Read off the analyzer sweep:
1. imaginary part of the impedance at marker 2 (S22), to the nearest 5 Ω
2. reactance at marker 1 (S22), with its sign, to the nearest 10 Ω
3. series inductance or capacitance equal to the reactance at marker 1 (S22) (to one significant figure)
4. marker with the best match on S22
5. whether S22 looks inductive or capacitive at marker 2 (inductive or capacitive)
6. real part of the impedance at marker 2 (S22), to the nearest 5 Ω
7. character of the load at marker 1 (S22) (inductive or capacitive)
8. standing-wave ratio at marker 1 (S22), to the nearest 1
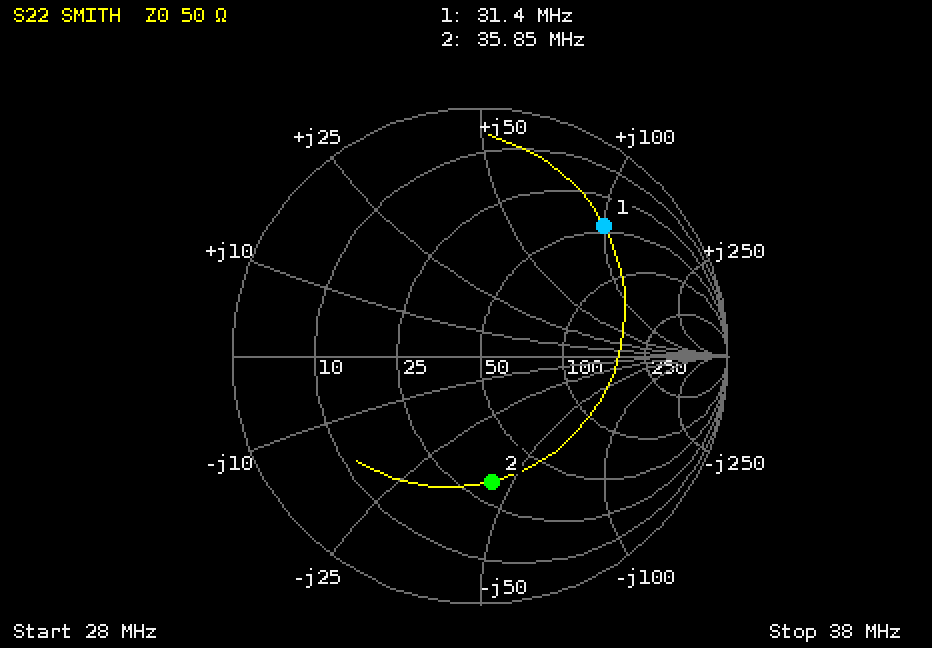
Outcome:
-45 Ω
+100 Ω
500 nH
marker 2
capacitive
30 Ω
inductive
6
